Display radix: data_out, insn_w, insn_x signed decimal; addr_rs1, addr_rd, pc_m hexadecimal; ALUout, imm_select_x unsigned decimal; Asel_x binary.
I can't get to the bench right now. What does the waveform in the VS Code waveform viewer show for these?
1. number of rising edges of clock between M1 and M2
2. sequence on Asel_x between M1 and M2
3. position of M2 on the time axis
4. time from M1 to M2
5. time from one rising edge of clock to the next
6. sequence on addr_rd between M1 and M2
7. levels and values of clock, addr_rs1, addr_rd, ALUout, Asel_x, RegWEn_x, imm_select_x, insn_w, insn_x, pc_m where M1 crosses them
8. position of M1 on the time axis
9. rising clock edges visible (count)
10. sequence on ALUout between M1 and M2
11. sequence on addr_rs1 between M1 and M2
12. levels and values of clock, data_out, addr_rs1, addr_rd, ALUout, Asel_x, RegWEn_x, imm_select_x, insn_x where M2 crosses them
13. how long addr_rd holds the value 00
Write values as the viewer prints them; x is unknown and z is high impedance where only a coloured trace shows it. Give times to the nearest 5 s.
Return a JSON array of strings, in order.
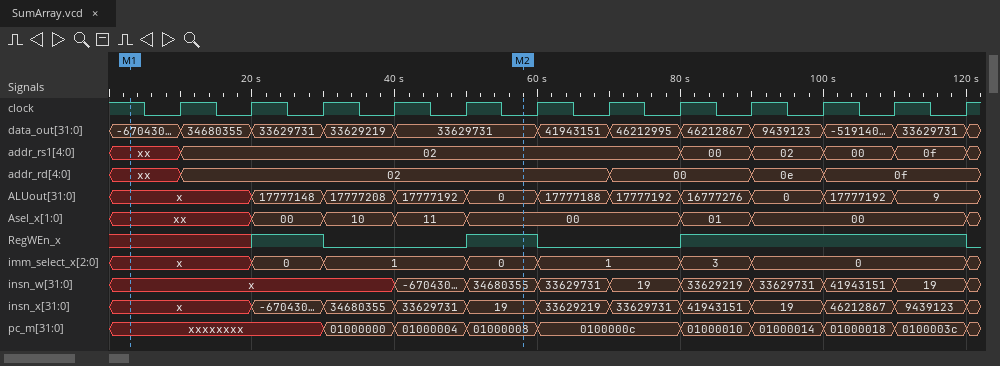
["5", "xx, 00, 10, 11, 00", "60 s", "55 s", "10 s", "xx, 02", "clock=1, addr_rs1=xx, addr_rd=xx, ALUout=x, Asel_x=xx, RegWEn_x=x, imm_select_x=x, insn_w=x, insn_x=x, pc_m=xxxxxxxx", "5 s", "12", "x, 17777148, 17777208, 17777192, 0", "xx, 02", "clock=0, data_out=33629731, addr_rs1=02, addr_rd=02, ALUout=0, Asel_x=00, RegWEn_x=1, imm_select_x=0, insn_x=19", "20 s"]
